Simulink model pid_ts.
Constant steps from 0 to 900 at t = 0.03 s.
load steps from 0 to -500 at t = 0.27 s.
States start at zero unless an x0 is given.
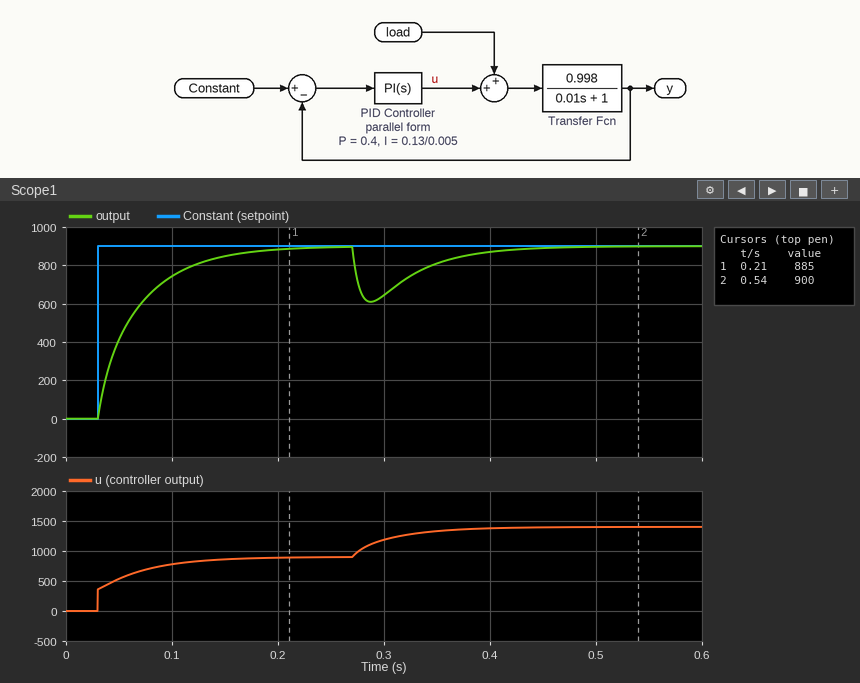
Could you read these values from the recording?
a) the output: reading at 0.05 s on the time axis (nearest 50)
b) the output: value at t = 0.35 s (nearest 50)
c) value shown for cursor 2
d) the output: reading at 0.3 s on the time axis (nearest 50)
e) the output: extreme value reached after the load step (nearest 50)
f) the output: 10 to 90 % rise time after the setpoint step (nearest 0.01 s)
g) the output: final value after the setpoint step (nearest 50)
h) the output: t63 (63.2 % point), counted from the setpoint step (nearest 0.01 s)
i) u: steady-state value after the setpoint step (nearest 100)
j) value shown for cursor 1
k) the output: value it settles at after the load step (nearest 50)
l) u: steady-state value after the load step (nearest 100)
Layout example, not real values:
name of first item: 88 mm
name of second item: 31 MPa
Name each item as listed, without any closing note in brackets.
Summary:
the output: reading at 0.05 s on the time axis: 400
the output: value at t = 0.35 s: 800
value shown for cursor 2: 900
the output: reading at 0.3 s on the time axis: 650
the output: extreme value reached after the load step: 600
the output: 10 to 90 % rise time after the setpoint step: 0.09 s
the output: final value after the setpoint step: 900
the output: t63 (63.2 % point), counted from the setpoint step: 0.04 s
u: steady-state value after the setpoint step: 900
value shown for cursor 1: 885
the output: value it settles at after the load step: 900
u: steady-state value after the load step: 1400
